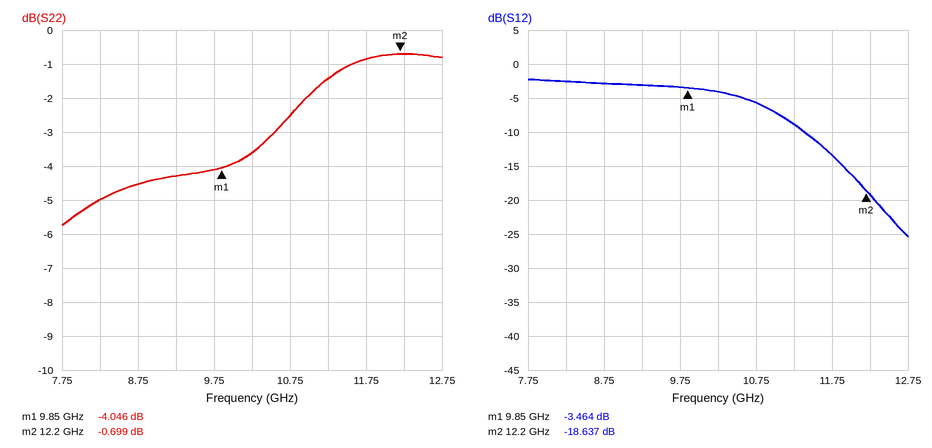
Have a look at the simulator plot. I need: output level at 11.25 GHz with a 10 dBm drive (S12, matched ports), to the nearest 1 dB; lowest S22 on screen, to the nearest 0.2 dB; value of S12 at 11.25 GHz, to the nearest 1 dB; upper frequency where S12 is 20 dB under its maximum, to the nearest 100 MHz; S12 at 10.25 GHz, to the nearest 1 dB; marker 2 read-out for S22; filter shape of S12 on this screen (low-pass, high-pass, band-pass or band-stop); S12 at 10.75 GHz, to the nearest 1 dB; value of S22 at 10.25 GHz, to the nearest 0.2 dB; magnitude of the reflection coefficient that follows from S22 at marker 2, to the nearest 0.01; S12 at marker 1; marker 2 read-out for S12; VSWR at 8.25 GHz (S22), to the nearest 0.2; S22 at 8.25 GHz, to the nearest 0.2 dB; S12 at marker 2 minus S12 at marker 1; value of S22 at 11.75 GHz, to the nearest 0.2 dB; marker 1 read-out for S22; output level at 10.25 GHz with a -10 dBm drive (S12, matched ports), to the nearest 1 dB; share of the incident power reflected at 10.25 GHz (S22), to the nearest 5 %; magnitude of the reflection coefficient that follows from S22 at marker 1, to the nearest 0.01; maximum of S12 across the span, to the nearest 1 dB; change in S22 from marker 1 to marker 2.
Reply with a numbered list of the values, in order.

1. 1 dBm
2. -5.8 dB
3. -9 dB
4. 12.5 GHz
5. -4 dB
6. -0.699 dB
7. low-pass
8. -6 dB
9. -3.6 dB
10. 0.92
11. -3.464 dB
12. -18.637 dB
13. 3.6
14. -5.0 dB
15. -15.173 dB
16. -0.8 dB
17. -4.046 dB
18. -14 dBm
19. 45 %
20. 0.63
21. -2 dB
22. 3.347 dB
